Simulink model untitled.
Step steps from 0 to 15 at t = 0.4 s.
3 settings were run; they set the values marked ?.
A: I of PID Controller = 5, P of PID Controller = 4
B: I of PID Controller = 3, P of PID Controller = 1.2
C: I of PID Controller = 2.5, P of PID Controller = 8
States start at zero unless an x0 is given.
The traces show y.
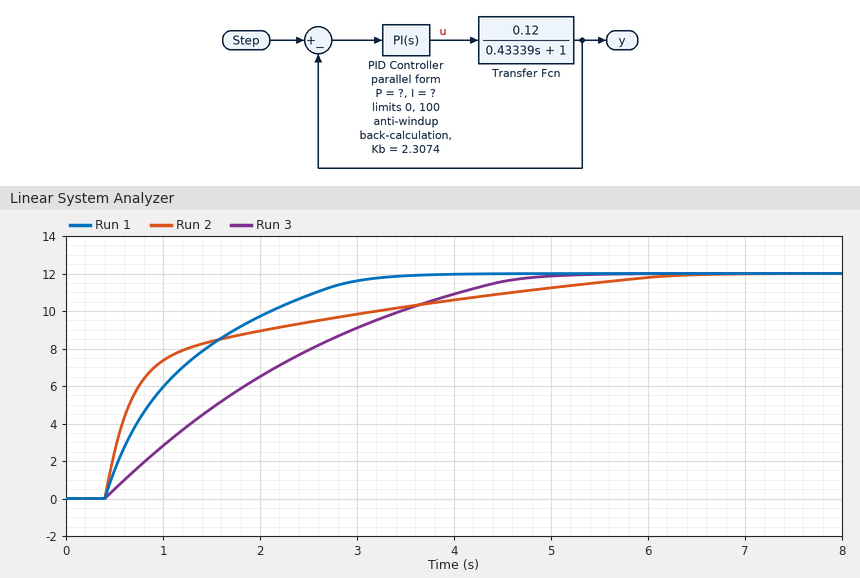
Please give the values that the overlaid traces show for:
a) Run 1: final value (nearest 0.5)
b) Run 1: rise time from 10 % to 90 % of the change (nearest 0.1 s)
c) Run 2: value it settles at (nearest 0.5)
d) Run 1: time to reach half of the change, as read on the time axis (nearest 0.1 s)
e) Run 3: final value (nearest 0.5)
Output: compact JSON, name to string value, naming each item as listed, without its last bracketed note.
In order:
{"Run 1: final value": "12.0", "Run 1: rise time from 10 % to 90 % of the change": "2.0 s", "Run 2: value it settles at": "12.0", "Run 1: time to reach half of the change, as read on the time axis": "1.0 s", "Run 3: final value": "12.0"}
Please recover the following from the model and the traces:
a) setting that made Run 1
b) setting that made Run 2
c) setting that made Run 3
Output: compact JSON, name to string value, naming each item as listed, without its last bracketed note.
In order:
{"setting that made Run 1": "A", "setting that made Run 2": "C", "setting that made Run 3": "B"}
